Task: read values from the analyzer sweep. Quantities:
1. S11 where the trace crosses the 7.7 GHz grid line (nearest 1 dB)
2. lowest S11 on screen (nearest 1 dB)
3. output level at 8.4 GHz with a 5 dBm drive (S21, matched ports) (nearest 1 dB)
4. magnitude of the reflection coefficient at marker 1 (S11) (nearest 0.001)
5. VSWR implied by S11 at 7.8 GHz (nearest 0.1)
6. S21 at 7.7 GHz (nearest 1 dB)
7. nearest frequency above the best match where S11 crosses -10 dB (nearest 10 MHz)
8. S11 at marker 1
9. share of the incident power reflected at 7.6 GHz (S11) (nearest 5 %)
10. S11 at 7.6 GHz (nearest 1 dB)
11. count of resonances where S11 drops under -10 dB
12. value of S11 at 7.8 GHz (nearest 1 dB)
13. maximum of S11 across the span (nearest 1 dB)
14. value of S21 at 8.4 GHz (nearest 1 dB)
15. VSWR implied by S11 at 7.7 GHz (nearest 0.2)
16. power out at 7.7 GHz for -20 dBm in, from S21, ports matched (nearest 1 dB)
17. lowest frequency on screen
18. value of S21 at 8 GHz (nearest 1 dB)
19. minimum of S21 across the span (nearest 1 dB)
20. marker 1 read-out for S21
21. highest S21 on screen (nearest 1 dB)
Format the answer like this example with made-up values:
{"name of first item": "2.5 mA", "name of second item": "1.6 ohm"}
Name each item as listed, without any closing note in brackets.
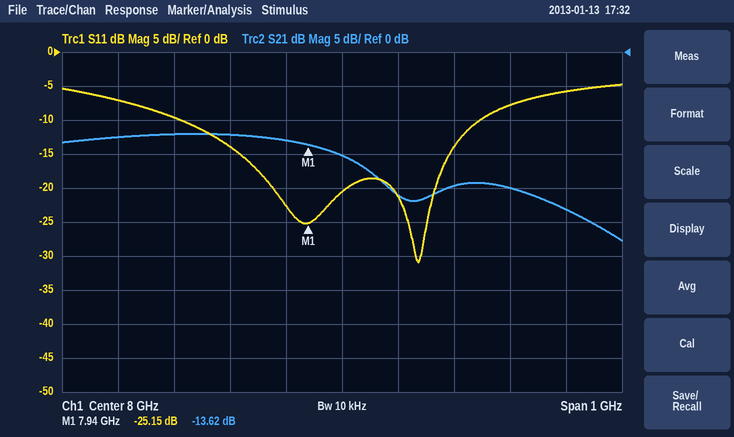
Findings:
{"S11 where the trace crosses the 7.7 GHz grid line": "-10 dB", "lowest S11 on screen": "-31 dB", "output level at 8.4 GHz with a 5 dBm drive (S21, matched ports)": "-18 dBm", "magnitude of the reflection coefficient at marker 1 (S11)": "0.055", "VSWR implied by S11 at 7.8 GHz": "1.5", "S21 at 7.7 GHz": "-12 dB", "nearest frequency above the best match where S11 crosses -10 dB": "8.25 GHz", "S11 at marker 1": "-25.15 dB", "share of the incident power reflected at 7.6 GHz (S11)": "20 %", "S11 at 7.6 GHz": "-7 dB", "count of resonances where S11 drops under -10 dB": "2", "value of S11 at 7.8 GHz": "-14 dB", "maximum of S11 across the span": "-5 dB", "value of S21 at 8.4 GHz": "-23 dB", "VSWR implied by S11 at 7.7 GHz": "2.0", "power out at 7.7 GHz for -20 dBm in, from S21, ports matched": "-32 dBm", "lowest frequency on screen": "7.5 GHz", "value of S21 at 8 GHz": "-15 dB", "minimum of S21 across the span": "-28 dB", "marker 1 read-out for S21": "-13.62 dB", "highest S21 on screen": "-12 dB"}
